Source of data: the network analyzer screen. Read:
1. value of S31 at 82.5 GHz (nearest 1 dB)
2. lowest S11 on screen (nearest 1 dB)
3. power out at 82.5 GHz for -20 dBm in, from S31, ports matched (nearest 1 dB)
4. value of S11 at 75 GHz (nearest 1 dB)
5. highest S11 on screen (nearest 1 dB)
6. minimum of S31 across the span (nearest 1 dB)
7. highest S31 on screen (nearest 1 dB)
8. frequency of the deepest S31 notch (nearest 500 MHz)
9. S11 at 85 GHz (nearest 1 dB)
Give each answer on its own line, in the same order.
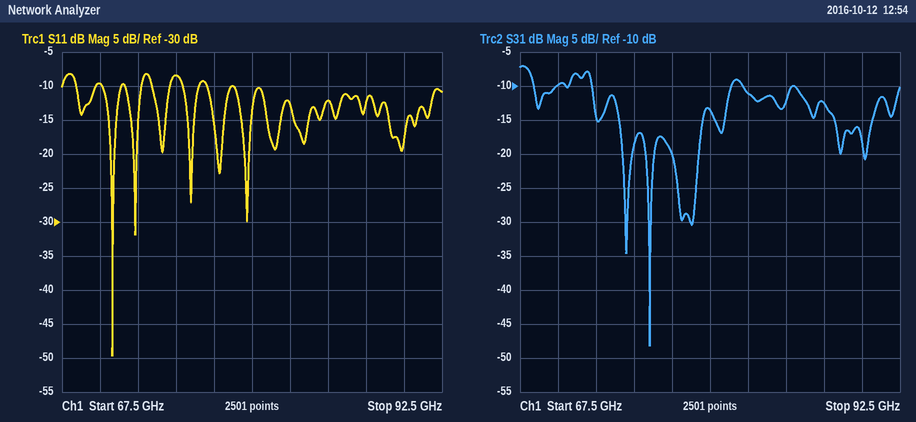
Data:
-11 dB
-50 dB
-31 dBm
-8 dB
-8 dB
-48 dB
-7 dB
76.0 GHz
-12 dB
